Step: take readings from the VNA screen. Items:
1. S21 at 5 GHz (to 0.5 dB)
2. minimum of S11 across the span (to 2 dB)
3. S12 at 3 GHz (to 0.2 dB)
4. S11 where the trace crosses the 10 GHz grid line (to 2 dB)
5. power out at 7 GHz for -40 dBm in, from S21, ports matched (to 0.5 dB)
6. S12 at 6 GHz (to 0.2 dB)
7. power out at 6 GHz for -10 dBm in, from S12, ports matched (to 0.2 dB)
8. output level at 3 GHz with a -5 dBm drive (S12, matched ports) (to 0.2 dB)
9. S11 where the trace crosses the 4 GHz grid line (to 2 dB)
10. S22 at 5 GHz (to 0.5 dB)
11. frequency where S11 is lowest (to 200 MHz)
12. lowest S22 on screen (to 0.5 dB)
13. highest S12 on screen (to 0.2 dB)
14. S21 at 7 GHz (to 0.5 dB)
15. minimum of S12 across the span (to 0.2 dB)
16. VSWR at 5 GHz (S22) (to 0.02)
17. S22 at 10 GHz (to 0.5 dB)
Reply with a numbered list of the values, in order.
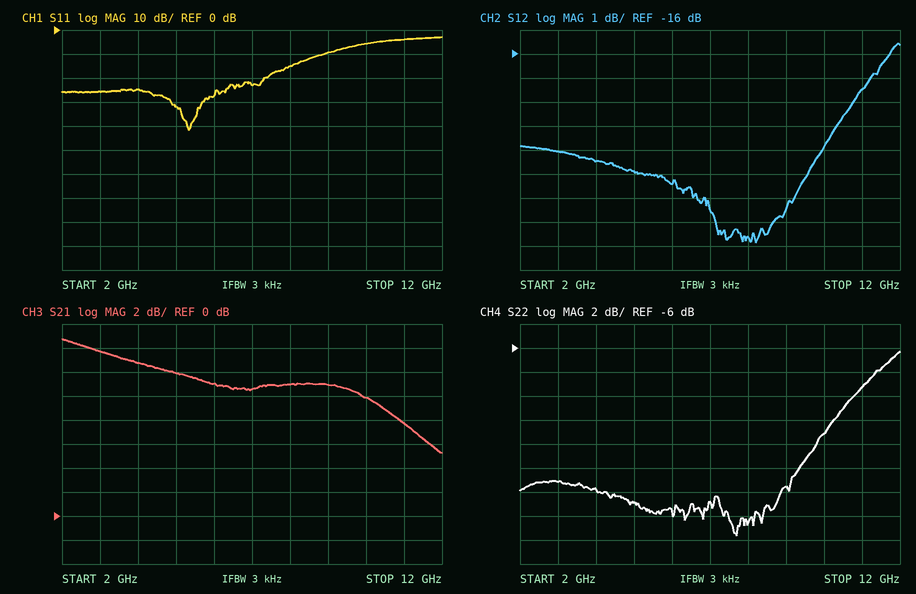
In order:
1. 12.0 dB
2. -42 dB
3. -20.0 dB
4. -6 dB
5. -29.5 dBm
6. -21.4 dB
7. -31.4 dBm
8. -25.0 dBm
9. -24 dB
10. -19.0 dB
11. 5.4 GHz
12. -21.5 dB
13. -15.6 dB
14. 10.5 dB
15. -23.8 dB
16. 1.26
17. -13.0 dB
